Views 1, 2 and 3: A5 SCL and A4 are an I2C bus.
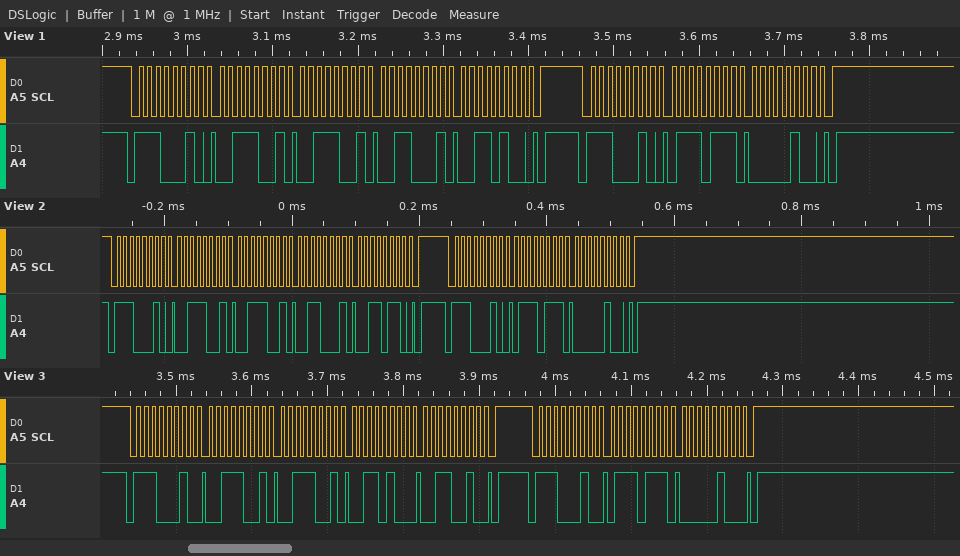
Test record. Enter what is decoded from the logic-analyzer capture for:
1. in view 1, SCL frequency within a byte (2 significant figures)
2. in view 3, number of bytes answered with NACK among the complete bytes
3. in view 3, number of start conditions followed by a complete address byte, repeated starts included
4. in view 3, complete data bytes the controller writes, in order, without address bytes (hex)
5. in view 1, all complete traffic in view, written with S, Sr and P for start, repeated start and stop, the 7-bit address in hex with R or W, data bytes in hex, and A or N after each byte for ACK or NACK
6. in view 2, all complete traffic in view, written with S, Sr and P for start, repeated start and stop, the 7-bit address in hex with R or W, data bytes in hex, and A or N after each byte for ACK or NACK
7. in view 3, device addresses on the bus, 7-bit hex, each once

100 kHz
0
2
39 39 34 32 77 04
S 71W A 39 A 39 A 31 A 34 A P S 71W A 77 A 04 A P
S 71W A 39 A 39 A 31 A 36 A P S 71W A 77 A 04 A P
0x71
